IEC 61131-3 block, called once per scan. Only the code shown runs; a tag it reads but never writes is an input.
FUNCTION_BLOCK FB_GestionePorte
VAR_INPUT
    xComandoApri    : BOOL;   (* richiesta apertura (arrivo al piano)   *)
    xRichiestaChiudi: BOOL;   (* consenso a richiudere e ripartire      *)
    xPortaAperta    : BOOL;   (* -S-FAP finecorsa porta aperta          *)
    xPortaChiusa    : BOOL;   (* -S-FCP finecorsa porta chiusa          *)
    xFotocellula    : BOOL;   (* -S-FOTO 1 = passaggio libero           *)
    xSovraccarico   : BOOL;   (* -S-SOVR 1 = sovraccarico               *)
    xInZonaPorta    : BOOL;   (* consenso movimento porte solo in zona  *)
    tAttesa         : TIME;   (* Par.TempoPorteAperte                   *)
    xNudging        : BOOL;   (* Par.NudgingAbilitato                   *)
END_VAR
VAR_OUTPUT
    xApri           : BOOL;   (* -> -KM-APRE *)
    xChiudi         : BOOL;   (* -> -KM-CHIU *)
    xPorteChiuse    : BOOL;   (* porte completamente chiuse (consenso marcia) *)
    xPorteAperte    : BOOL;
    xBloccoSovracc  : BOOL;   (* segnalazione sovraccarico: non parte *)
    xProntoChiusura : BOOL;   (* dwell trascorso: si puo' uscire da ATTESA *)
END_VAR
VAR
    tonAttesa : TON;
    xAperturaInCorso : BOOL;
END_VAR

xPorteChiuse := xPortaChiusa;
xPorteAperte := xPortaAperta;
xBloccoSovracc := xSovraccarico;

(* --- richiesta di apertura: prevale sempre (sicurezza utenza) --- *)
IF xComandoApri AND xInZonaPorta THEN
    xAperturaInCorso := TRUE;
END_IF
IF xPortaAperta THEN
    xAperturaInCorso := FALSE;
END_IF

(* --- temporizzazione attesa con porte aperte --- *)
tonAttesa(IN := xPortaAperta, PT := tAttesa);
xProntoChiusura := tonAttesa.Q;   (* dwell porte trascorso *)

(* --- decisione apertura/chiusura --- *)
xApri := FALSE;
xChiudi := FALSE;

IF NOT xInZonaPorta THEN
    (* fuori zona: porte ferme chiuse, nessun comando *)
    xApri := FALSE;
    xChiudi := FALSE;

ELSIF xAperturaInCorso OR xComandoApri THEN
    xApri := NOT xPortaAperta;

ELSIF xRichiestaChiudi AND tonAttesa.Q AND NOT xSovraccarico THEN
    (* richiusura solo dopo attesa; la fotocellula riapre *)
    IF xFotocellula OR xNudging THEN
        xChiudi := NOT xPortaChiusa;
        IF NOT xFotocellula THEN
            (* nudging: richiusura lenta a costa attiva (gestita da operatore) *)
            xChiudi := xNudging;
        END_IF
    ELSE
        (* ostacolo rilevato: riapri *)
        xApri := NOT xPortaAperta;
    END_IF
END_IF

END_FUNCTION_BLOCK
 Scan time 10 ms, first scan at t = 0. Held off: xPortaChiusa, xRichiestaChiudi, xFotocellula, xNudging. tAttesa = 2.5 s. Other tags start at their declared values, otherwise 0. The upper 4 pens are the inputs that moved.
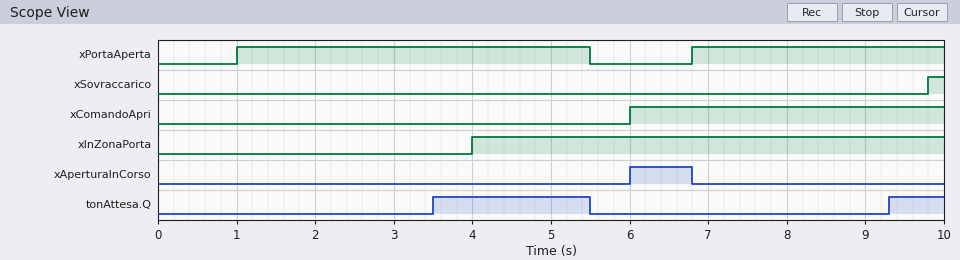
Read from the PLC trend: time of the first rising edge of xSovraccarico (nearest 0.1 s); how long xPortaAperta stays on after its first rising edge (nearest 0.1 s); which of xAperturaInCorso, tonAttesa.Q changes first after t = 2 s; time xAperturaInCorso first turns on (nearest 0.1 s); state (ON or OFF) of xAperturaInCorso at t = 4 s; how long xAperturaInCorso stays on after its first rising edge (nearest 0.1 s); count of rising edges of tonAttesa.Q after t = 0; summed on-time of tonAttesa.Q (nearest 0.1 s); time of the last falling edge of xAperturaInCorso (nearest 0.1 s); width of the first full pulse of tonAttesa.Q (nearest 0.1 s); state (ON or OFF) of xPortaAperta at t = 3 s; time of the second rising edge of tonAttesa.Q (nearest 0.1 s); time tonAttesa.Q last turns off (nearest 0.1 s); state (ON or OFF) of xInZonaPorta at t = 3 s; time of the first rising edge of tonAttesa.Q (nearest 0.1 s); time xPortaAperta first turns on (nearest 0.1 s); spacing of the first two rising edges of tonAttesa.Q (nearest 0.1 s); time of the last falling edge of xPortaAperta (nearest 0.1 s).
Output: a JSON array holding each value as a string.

["9.8 s", "4.5 s", "tonAttesa.Q", "6.0 s", "OFF", "0.8 s", "2", "2.7 s", "6.8 s", "2.0 s", "ON", "9.3 s", "5.5 s", "OFF", "3.5 s", "1.0 s", "5.8 s", "5.5 s"]
